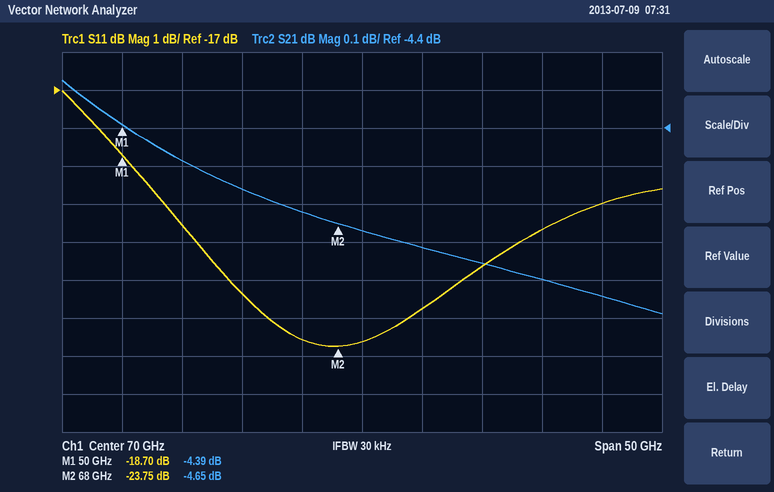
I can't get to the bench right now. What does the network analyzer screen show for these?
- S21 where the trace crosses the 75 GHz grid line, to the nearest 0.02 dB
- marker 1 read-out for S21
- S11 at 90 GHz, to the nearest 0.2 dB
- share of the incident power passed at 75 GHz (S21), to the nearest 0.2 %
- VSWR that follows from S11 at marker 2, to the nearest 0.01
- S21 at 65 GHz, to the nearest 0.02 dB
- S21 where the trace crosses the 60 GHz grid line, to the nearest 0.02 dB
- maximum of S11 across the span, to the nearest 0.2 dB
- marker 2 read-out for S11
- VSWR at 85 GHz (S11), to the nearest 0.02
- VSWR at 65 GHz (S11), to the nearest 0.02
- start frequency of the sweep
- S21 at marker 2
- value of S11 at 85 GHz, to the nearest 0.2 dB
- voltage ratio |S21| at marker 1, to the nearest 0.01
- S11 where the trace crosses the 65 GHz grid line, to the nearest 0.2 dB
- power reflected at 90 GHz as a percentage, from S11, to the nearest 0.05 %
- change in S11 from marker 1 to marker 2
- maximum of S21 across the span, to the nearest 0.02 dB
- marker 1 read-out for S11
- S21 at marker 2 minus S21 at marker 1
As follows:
-4.72 dB
-4.39 dB
-20.0 dB
33.8 %
1.14
-4.62 dB
-4.56 dB
-17.0 dB
-23.75 dB
1.20
1.14
45 GHz
-4.65 dB
-20.6 dB
0.60
-23.6 dB
1.00 %
-5.05 dB
-4.28 dB
-18.70 dB
-0.26 dB
